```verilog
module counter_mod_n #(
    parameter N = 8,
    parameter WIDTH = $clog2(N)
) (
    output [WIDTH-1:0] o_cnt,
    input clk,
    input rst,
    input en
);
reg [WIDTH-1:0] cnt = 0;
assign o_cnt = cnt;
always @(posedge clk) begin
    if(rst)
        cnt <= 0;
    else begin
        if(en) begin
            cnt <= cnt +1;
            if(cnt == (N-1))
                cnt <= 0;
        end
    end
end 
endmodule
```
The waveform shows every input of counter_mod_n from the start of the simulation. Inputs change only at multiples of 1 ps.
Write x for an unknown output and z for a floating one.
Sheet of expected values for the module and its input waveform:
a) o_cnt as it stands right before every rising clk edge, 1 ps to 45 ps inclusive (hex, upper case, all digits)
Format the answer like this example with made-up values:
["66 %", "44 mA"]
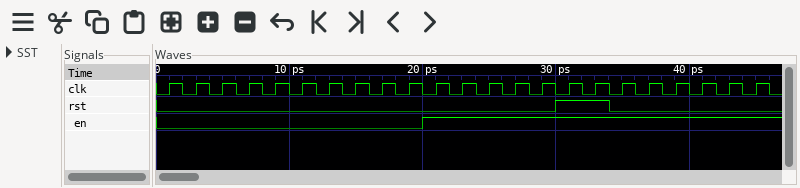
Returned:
["0, 0, 0, 0, 0, 0, 0, 0, 0, 0, 0, 1, 2, 3, 4, 5, 0, 0, 1, 2, 3, 4, 5"]
